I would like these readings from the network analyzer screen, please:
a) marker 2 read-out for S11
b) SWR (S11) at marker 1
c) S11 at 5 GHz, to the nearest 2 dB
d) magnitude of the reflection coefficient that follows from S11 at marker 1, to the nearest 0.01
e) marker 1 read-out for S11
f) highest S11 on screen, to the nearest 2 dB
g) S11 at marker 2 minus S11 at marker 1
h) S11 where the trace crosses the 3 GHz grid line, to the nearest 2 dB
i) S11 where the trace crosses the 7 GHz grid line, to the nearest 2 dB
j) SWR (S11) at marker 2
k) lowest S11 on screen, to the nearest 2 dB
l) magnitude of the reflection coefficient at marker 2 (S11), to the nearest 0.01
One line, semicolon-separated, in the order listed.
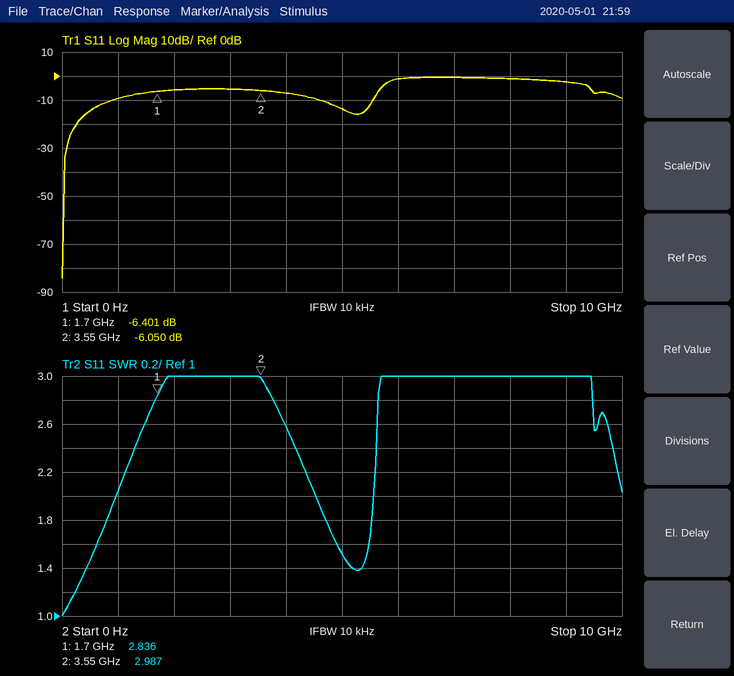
-6.050 dB; 2.836; -14 dB; 0.48; -6.401 dB; 0 dB; 0.351 dB; -6 dB; 0 dB; 2.987; -84 dB; 0.50
